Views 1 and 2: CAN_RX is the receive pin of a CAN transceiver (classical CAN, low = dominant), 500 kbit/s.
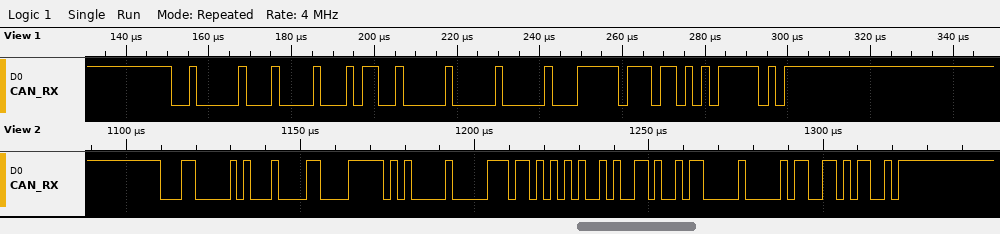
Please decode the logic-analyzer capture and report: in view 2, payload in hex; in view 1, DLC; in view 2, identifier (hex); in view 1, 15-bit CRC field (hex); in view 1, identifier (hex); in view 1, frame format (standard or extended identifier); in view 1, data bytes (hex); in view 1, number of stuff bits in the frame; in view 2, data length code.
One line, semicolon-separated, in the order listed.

61 FA 00 6D 54 A6 96 00; 4; 0x181; 0x6D5F; 0x201; standard; 59 00 00 3F; 6; 8
